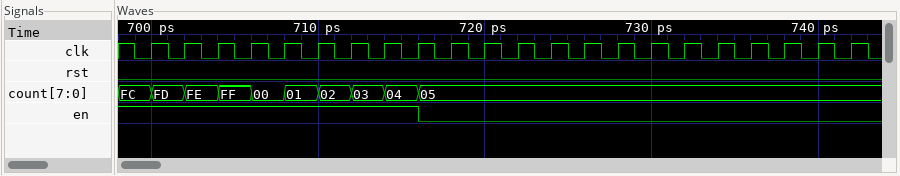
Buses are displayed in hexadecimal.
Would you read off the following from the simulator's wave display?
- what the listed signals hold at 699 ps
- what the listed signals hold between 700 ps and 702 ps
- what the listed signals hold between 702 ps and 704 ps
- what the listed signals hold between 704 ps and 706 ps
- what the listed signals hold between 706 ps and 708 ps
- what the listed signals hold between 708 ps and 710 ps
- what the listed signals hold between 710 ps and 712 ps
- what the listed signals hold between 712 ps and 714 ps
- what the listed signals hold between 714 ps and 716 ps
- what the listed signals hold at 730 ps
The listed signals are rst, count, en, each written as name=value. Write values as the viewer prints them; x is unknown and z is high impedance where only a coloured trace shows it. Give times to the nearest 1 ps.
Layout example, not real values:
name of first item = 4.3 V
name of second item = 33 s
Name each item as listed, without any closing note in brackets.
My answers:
what the listed signals hold at 699 ps = rst=0, count=FC, en=1
what the listed signals hold between 700 ps and 702 ps = rst=0, count=FD, en=1
what the listed signals hold between 702 ps and 704 ps = rst=0, count=FE, en=1
what the listed signals hold between 704 ps and 706 ps = rst=0, count=FF, en=1
what the listed signals hold between 706 ps and 708 ps = rst=0, count=00, en=1
what the listed signals hold between 708 ps and 710 ps = rst=0, count=01, en=1
what the listed signals hold between 710 ps and 712 ps = rst=0, count=02, en=1
what the listed signals hold between 712 ps and 714 ps = rst=0, count=03, en=1
what the listed signals hold between 714 ps and 716 ps = rst=0, count=04, en=1
what the listed signals hold at 730 ps = rst=0, count=05, en=0
